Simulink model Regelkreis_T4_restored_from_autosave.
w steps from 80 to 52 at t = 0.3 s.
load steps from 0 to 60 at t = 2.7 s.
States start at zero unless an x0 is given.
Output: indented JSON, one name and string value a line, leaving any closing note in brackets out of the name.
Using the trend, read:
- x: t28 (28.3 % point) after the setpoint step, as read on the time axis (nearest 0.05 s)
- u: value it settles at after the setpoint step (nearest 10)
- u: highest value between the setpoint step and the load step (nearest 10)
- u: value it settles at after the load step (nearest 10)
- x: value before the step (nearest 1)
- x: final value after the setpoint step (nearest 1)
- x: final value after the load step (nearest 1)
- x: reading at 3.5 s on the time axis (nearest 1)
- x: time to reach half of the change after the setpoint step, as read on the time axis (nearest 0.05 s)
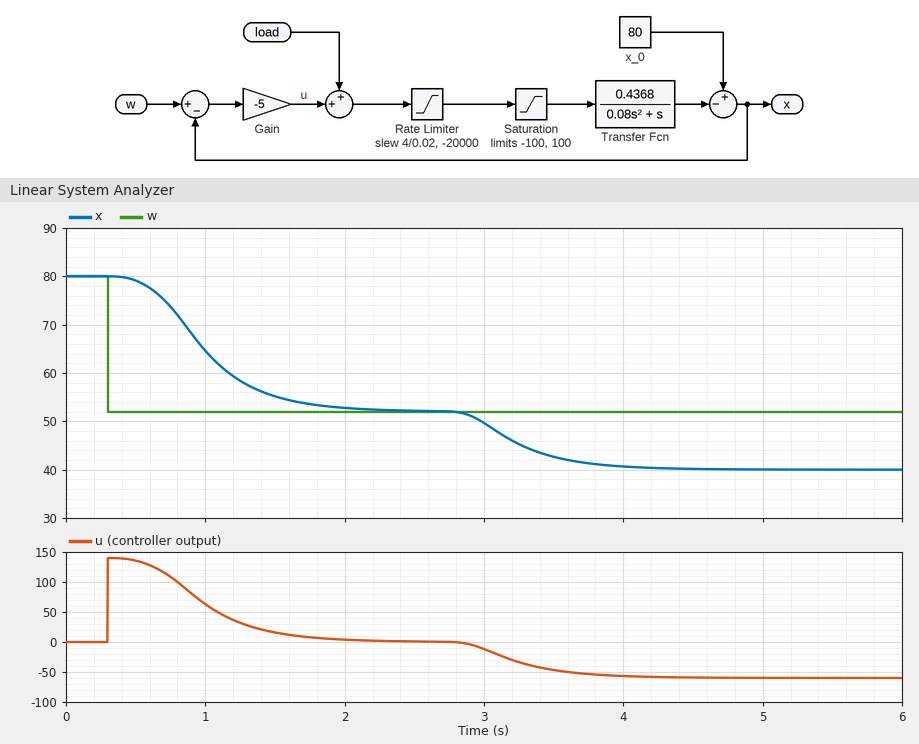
{
  "x: t28 (28.3 % point) after the setpoint step, as read on the time axis": "0.80 s",
  "u: value it settles at after the setpoint step": "0",
  "u: highest value between the setpoint step and the load step": "140",
  "u: value it settles at after the load step": "-60",
  "x: value before the step": "80",
  "x: final value after the setpoint step": "52",
  "x: final value after the load step": "40",
  "x: reading at 3.5 s on the time axis": "43",
  "x: time to reach half of the change after the setpoint step, as read on the time axis": "0.95 s"
}
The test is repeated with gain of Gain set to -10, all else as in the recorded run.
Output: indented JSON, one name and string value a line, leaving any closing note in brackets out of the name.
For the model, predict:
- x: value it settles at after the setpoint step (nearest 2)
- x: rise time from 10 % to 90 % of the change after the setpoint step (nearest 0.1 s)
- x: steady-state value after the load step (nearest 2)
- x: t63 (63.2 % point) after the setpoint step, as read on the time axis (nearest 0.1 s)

{
  "x: value it settles at after the setpoint step": "52",
  "x: rise time from 10 % to 90 % of the change after the setpoint step": "0.6 s",
  "x: steady-state value after the load step": "46",
  "x: t63 (63.2 % point) after the setpoint step, as read on the time axis": "1.0 s"
}
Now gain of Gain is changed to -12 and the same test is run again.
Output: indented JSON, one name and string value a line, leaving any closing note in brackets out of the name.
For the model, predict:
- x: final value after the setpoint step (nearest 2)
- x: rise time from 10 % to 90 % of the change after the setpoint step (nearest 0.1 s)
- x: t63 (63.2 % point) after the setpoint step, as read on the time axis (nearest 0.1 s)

{
  "x: final value after the setpoint step": "52",
  "x: rise time from 10 % to 90 % of the change after the setpoint step": "0.6 s",
  "x: t63 (63.2 % point) after the setpoint step, as read on the time axis": "1.0 s"
}
